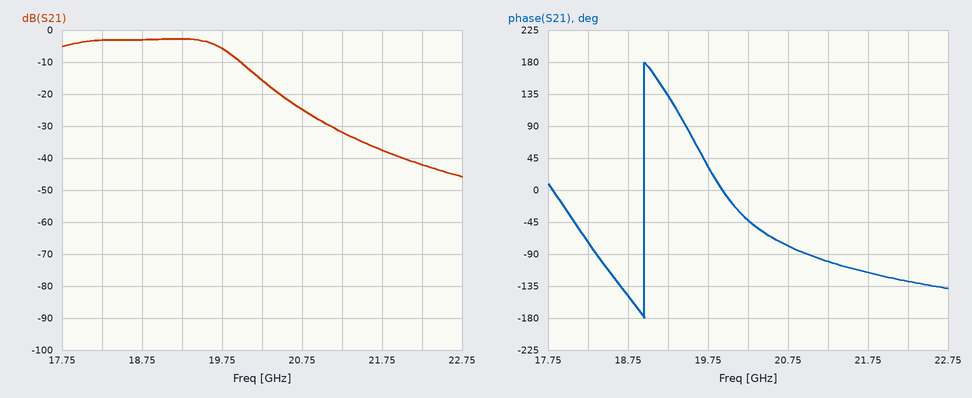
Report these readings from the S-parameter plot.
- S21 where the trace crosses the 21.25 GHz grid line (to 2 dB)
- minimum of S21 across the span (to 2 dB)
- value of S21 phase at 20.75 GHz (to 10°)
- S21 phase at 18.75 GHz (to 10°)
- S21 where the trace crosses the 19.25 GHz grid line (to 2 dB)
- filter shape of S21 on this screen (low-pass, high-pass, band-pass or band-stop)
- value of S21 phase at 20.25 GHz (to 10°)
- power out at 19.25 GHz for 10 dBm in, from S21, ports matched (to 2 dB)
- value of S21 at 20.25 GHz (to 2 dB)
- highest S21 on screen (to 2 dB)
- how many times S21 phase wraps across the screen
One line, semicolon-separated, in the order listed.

-32 dB; -46 dB; -80°; -150°; -2 dB; low-pass; -40°; 8 dBm; -16 dB; -2 dB; 1
